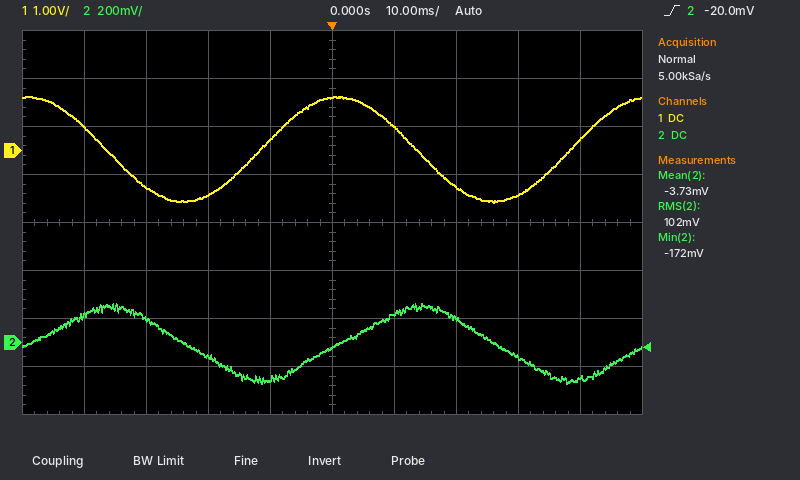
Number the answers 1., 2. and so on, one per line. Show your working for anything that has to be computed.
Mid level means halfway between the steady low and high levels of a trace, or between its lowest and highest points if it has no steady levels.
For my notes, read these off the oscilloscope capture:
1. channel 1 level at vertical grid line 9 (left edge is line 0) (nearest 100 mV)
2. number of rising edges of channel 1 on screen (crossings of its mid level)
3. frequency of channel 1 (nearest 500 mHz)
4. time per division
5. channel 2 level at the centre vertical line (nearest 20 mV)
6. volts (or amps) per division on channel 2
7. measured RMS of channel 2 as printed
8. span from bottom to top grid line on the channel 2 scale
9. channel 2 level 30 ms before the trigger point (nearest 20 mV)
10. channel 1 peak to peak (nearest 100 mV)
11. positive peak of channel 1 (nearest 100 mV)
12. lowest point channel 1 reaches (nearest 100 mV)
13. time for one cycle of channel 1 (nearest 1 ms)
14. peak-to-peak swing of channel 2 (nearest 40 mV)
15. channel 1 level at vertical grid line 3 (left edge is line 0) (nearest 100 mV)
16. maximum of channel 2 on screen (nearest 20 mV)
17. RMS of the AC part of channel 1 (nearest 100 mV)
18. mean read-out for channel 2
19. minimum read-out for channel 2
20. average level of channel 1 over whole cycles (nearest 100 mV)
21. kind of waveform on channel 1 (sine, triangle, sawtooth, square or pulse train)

1. 200 mV
2. 2
3. 1 / 50 ms ≈ 20.0 Hz
4. 10 ms
5. -20 mV
6. 200 mV
7. 102 mV
8. 1.6 V
9. 100 mV
10. 1.1 V − (-1.1 V) = 2.2 V
11. 1.1 V
12. -1.1 V
13. 50 ms
14. 320 mV
15. -900 mV
16. 160 mV
17. 2.2 V / (2√2) ≈ 778 mV, so 800 mV to the nearest 100 mV
18. -3.73 mV
19. -172 mV
20. (1.1 V + (-1.1 V)) / 2 ≈ 0.0 V
21. sine
